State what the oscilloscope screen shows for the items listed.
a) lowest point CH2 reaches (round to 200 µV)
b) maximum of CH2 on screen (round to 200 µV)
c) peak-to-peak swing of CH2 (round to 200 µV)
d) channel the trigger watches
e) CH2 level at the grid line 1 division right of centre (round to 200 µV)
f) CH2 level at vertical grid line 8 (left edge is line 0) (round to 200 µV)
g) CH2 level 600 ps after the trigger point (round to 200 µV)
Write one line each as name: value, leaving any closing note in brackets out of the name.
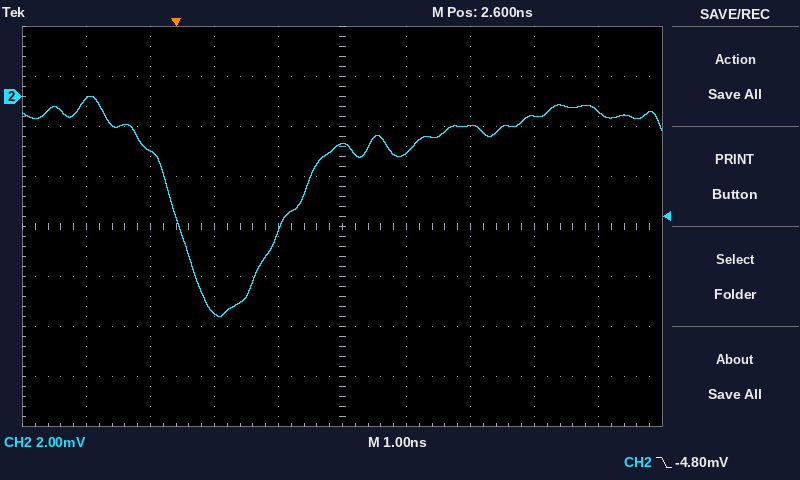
lowest point CH2 reaches: -8.8 mV
maximum of CH2 on screen: 0.0 mV
peak-to-peak swing of CH2: 8.8 mV
channel the trigger watches: CH2
CH2 level at the grid line 1 division right of centre: -2.2 mV
CH2 level at vertical grid line 8 (left edge is line 0): -800 µV
CH2 level 600 ps after the trigger point: -8.6 mV
